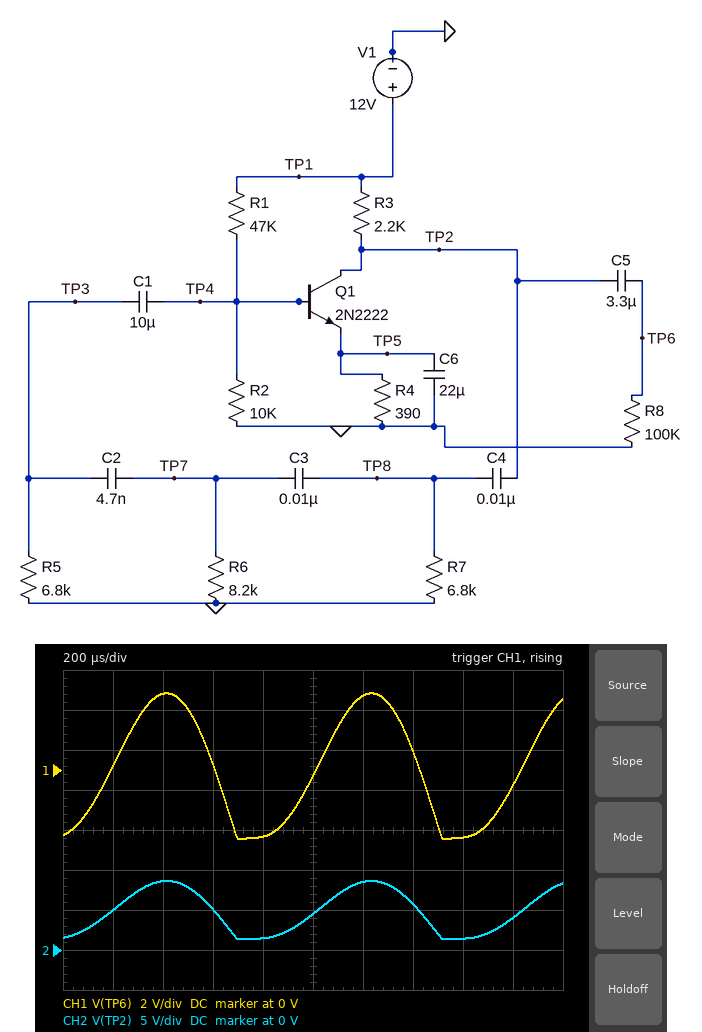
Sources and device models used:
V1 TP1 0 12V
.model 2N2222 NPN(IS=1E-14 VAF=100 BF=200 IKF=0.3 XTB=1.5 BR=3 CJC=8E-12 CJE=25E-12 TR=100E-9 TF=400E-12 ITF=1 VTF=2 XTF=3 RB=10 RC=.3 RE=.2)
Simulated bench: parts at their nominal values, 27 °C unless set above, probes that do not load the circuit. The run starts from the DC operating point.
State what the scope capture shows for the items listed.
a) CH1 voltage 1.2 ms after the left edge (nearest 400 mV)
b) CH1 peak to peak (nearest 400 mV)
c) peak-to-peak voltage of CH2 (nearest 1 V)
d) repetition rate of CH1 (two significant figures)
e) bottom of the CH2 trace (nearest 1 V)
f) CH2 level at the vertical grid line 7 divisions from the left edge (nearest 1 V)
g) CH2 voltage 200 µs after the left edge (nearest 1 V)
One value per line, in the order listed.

3.6 V
7.2 V
7 V
1.2 kHz
1 V
6 V
5 V
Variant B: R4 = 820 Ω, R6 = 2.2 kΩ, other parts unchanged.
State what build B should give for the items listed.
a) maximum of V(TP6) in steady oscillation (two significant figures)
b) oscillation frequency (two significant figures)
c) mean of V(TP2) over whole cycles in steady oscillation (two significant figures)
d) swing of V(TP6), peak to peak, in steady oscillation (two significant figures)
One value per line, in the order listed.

3.2 V
2.0 kHz
8.3 V
6.4 V
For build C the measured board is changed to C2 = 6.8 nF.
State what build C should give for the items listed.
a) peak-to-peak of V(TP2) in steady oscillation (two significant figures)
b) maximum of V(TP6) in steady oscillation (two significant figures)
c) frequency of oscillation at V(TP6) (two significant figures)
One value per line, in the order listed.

7.4 V
4.0 V
1.1 kHz
